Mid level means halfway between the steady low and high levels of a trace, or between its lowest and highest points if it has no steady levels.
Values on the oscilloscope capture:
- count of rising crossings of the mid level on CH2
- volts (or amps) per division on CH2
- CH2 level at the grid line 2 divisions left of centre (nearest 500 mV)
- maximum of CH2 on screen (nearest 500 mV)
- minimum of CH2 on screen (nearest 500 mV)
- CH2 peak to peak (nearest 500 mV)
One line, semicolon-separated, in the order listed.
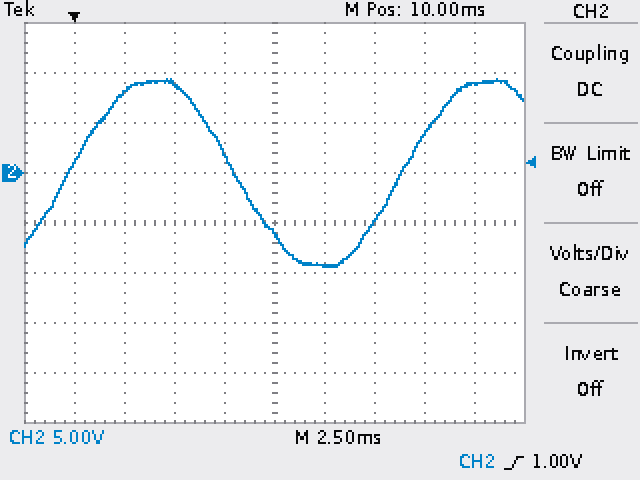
2; 5 V; 9.0 V; 9.5 V; -9.5 V; 19.0 V
